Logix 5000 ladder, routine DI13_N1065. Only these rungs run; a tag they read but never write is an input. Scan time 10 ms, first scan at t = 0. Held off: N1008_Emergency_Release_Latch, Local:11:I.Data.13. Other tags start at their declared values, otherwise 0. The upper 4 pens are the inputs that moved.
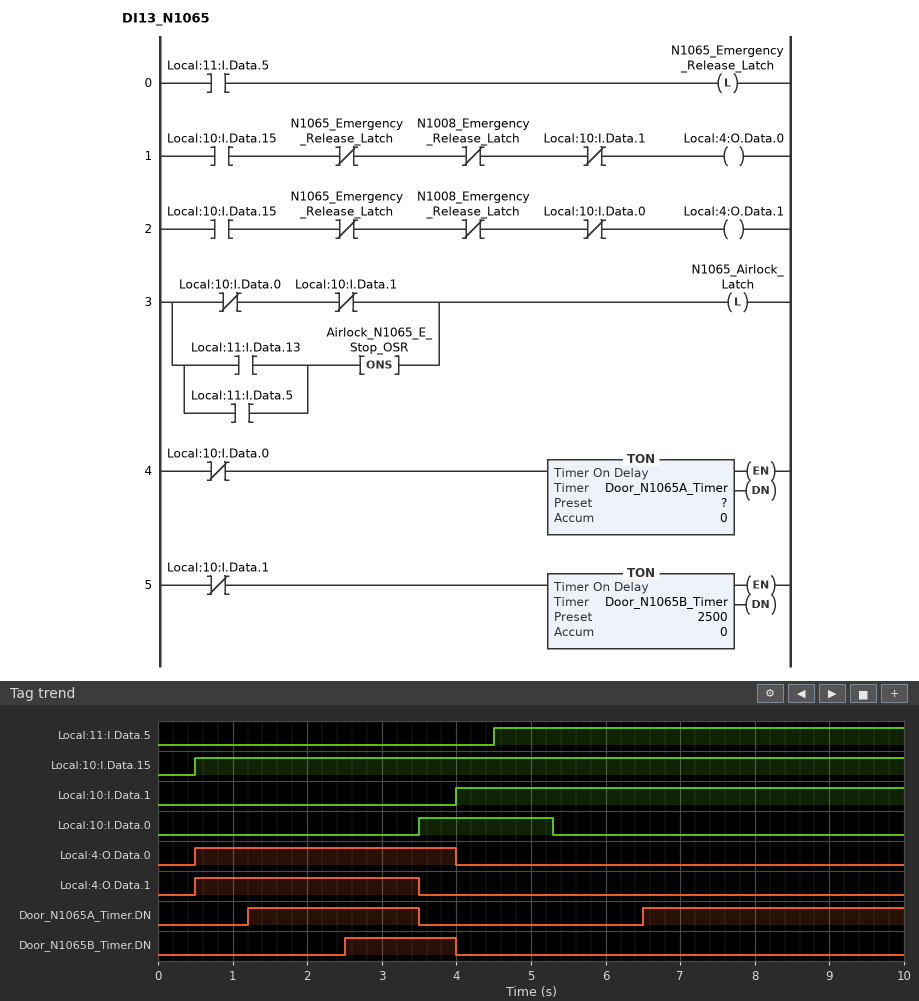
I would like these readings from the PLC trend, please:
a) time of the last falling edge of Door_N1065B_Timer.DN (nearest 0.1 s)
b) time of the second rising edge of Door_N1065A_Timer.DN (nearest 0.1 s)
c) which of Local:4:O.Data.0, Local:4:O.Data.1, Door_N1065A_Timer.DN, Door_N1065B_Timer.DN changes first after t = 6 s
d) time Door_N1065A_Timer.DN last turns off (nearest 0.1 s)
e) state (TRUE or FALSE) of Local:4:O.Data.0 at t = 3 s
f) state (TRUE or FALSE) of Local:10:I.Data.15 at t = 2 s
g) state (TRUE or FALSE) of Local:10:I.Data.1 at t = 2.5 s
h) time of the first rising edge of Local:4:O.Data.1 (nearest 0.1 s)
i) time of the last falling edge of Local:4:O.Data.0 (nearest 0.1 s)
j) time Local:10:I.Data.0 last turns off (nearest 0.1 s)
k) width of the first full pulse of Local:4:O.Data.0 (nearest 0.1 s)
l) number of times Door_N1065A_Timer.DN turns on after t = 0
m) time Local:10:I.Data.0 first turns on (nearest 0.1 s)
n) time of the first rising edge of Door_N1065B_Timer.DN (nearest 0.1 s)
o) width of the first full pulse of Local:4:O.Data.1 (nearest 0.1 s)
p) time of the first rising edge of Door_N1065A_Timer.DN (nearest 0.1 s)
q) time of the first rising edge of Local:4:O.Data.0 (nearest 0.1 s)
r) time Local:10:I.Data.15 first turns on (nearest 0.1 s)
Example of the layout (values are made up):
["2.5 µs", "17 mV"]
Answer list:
["4.0 s", "6.5 s", "Door_N1065A_Timer.DN", "3.5 s", "TRUE", "TRUE", "FALSE", "0.5 s", "4.0 s", "5.3 s", "3.5 s", "2", "3.5 s", "2.5 s", "3.0 s", "1.2 s", "0.5 s", "0.5 s"]
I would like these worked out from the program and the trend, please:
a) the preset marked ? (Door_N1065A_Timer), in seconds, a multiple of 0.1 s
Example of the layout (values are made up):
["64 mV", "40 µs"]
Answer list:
["1.2 s"]
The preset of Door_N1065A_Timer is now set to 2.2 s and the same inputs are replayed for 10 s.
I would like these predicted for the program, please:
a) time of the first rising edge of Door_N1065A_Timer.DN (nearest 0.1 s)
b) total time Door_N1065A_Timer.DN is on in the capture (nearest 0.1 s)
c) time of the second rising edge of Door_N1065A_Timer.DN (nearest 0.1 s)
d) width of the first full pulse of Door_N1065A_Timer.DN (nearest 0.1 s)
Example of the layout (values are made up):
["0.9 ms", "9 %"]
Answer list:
["2.2 s", "3.8 s", "7.5 s", "1.3 s"]
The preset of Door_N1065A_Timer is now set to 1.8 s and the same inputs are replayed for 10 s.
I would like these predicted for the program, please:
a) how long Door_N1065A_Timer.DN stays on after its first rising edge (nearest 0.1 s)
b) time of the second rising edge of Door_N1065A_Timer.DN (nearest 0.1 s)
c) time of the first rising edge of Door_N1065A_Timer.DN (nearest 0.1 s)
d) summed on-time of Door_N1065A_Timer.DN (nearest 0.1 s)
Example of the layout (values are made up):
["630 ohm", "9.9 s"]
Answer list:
["1.7 s", "7.1 s", "1.8 s", "4.6 s"]
